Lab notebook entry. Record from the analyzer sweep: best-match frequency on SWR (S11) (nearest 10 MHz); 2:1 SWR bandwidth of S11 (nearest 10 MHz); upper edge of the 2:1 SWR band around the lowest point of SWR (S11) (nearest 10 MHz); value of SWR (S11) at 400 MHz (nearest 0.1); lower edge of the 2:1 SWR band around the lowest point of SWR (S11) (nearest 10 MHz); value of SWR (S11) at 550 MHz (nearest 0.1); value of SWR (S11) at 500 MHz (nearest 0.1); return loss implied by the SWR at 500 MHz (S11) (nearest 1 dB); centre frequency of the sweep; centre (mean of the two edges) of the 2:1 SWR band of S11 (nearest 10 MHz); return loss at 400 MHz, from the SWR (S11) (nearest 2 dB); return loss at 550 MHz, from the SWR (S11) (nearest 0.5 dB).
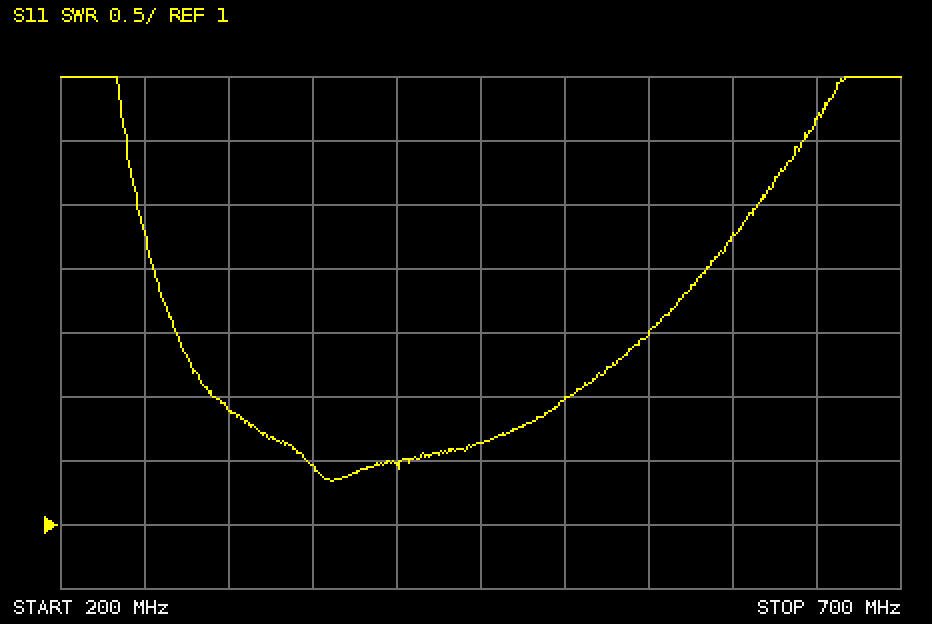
360 MHz
210 MHz
500 MHz
1.5
290 MHz
2.5
2.0
10 dB
450 MHz
400 MHz
14 dB
7.5 dB
